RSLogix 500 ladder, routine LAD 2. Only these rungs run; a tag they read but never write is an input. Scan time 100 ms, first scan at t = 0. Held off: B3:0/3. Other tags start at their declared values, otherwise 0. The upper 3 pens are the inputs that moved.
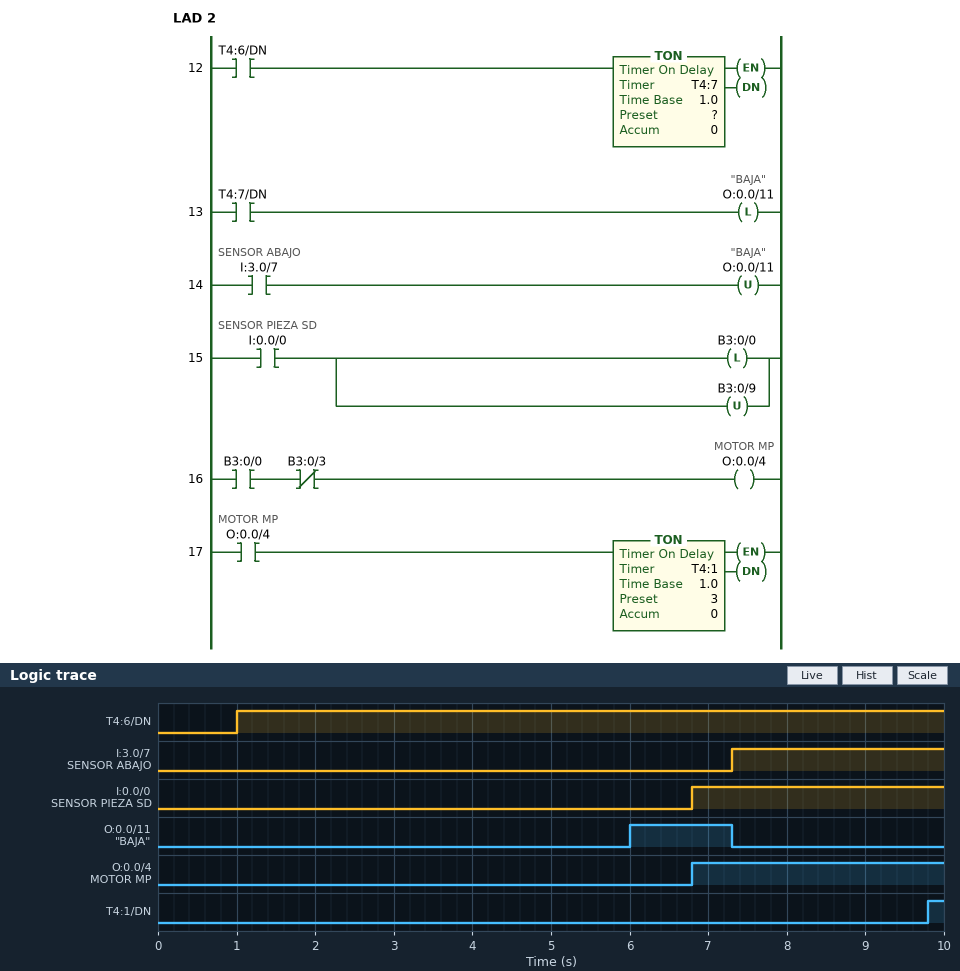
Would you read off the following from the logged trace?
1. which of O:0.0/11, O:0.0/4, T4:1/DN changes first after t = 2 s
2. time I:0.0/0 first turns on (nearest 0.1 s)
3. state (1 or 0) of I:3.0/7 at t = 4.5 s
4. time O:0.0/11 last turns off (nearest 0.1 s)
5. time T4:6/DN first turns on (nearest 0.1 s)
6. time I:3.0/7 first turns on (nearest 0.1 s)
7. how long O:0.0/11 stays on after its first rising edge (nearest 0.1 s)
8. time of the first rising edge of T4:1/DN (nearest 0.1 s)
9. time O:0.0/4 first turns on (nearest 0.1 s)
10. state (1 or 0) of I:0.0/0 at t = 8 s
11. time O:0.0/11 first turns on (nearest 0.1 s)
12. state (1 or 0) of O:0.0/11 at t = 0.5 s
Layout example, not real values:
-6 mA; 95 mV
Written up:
O:0.0/11; 6.8 s; 0; 7.3 s; 1.0 s; 7.3 s; 1.3 s; 9.8 s; 6.8 s; 1; 6.0 s; 0
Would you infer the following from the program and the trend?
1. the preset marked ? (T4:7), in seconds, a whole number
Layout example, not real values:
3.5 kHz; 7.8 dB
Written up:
5 s
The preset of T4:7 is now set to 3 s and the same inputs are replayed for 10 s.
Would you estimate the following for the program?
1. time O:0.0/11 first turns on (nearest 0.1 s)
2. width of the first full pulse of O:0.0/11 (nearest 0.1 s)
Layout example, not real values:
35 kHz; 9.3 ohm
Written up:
4.0 s; 3.3 s
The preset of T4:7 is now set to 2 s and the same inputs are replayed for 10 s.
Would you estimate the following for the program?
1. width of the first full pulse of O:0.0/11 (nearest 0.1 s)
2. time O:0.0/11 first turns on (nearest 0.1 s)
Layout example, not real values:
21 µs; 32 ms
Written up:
4.3 s; 3.0 s
